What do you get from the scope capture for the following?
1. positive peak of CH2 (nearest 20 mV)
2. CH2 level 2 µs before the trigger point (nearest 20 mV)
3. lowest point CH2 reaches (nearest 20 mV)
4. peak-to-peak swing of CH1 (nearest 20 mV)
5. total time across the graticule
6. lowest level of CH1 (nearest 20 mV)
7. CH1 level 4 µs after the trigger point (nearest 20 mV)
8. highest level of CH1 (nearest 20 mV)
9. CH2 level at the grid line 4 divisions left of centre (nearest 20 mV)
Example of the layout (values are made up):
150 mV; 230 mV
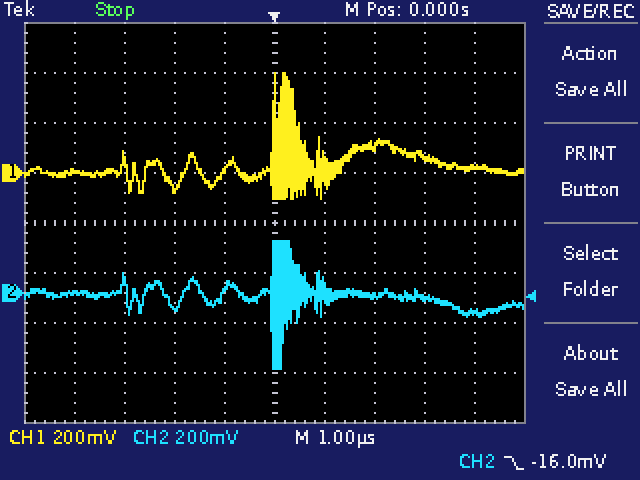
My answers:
200 mV; -60 mV; -300 mV; 500 mV; 10 µs; -100 mV; 20 mV; 400 mV; 0 mV
